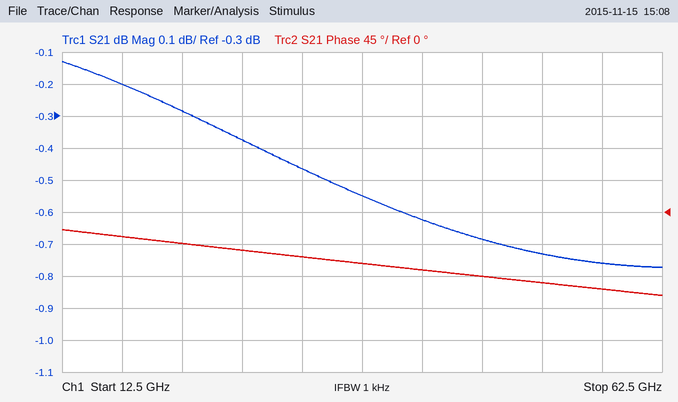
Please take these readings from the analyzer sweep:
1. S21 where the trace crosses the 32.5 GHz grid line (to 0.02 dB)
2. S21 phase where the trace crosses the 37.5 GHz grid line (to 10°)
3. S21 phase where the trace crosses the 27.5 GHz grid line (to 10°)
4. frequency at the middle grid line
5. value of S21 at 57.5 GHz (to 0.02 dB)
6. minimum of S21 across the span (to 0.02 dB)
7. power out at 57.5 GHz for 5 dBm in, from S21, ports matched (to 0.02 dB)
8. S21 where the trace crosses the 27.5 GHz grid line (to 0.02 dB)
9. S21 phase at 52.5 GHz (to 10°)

-0.46 dB
-70°
-50°
37.5 GHz
-0.76 dB
-0.78 dB
4.24 dBm
-0.38 dB
-100°
